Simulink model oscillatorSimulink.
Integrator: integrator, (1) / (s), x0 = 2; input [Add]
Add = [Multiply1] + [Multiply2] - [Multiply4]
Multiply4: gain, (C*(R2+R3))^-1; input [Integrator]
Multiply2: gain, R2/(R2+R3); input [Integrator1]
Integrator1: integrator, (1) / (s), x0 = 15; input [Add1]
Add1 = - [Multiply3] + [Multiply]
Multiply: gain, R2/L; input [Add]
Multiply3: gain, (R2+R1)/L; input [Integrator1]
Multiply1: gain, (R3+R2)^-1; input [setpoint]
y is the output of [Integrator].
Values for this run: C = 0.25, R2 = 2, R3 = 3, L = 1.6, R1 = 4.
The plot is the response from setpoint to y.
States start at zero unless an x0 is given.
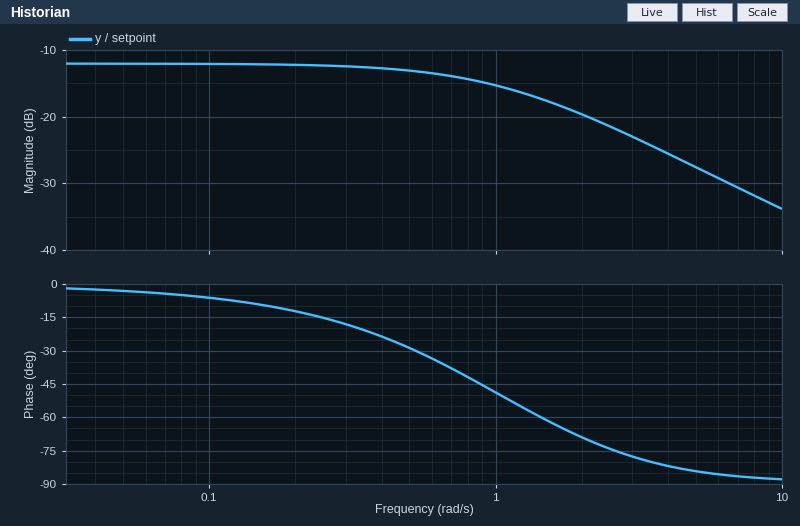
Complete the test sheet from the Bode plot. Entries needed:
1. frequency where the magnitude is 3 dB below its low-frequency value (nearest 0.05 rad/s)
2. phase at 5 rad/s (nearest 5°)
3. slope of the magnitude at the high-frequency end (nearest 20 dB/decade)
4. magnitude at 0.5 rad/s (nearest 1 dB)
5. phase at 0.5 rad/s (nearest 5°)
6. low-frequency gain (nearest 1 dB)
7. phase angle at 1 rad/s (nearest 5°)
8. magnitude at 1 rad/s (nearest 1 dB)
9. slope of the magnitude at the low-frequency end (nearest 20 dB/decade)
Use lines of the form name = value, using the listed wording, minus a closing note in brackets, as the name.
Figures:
frequency where the magnitude is 3 dB below its low-frequency value = 0.95 rad/s
phase at 5 rad/s = -85°
slope of the magnitude at the high-frequency end = -20 dB/decade
magnitude at 0.5 rad/s = -13 dB
phase at 0.5 rad/s = -30°
low-frequency gain = -12 dB
phase angle at 1 rad/s = -50°
magnitude at 1 rad/s = -15 dB
slope of the magnitude at the low-frequency end = 0 dB/decade
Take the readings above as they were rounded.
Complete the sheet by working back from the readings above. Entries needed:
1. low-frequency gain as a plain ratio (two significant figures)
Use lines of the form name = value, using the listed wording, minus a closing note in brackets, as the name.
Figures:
low-frequency gain as a plain ratio = 0.25
